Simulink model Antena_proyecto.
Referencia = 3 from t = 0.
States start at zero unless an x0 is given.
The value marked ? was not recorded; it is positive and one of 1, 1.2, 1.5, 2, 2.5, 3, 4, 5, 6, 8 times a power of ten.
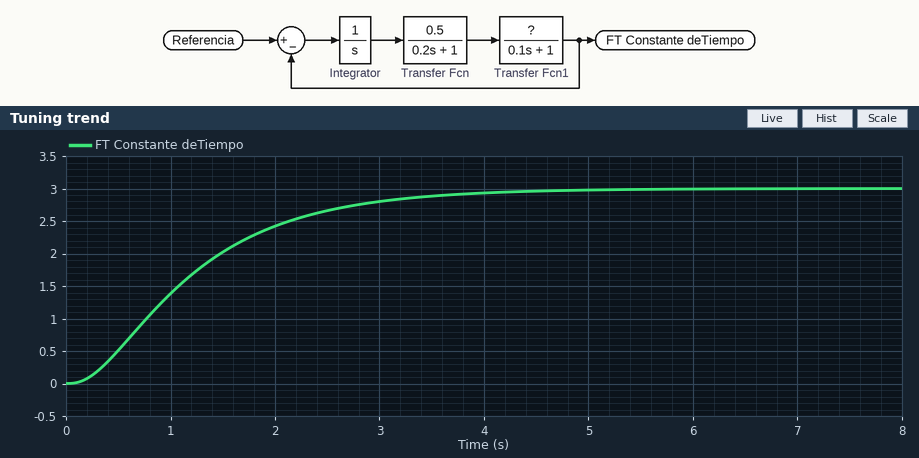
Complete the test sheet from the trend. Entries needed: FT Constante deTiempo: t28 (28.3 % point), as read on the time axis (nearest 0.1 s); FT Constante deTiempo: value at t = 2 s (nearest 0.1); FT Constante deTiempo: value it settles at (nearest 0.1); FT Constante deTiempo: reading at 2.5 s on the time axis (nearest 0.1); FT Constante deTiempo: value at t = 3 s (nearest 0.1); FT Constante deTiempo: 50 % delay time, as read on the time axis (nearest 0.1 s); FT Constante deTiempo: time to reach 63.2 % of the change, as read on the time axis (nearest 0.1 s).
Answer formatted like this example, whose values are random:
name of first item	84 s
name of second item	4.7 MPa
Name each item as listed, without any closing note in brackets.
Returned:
FT Constante deTiempo: t28 (28.3 % point), as read on the time axis	0.7 s
FT Constante deTiempo: value at t = 2 s	2.4
FT Constante deTiempo: value it settles at	3.0
FT Constante deTiempo: reading at 2.5 s on the time axis	2.7
FT Constante deTiempo: value at t = 3 s	2.8
FT Constante deTiempo: 50 % delay time, as read on the time axis	1.1 s
FT Constante deTiempo: time to reach 63.2 % of the change, as read on the time axis	1.4 s
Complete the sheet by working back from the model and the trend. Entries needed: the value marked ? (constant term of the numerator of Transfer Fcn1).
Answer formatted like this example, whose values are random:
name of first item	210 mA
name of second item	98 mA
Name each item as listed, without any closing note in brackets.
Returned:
the value marked ?	1.5
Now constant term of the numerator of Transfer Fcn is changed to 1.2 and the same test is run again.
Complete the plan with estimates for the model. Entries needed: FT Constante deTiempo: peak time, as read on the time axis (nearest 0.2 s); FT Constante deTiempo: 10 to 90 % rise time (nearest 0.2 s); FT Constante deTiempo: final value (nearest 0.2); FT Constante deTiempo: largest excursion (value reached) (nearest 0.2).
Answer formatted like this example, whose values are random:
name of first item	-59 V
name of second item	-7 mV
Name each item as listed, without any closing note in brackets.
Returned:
FT Constante deTiempo: peak time, as read on the time axis	1.6 s
FT Constante deTiempo: 10 to 90 % rise time	0.8 s
FT Constante deTiempo: final value	3.0
FT Constante deTiempo: largest excursion (value reached)	3.2
